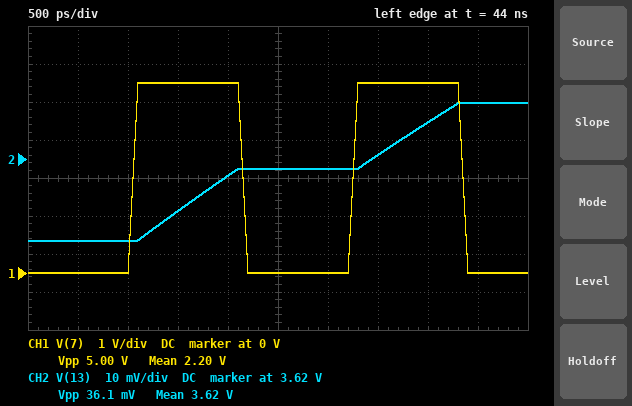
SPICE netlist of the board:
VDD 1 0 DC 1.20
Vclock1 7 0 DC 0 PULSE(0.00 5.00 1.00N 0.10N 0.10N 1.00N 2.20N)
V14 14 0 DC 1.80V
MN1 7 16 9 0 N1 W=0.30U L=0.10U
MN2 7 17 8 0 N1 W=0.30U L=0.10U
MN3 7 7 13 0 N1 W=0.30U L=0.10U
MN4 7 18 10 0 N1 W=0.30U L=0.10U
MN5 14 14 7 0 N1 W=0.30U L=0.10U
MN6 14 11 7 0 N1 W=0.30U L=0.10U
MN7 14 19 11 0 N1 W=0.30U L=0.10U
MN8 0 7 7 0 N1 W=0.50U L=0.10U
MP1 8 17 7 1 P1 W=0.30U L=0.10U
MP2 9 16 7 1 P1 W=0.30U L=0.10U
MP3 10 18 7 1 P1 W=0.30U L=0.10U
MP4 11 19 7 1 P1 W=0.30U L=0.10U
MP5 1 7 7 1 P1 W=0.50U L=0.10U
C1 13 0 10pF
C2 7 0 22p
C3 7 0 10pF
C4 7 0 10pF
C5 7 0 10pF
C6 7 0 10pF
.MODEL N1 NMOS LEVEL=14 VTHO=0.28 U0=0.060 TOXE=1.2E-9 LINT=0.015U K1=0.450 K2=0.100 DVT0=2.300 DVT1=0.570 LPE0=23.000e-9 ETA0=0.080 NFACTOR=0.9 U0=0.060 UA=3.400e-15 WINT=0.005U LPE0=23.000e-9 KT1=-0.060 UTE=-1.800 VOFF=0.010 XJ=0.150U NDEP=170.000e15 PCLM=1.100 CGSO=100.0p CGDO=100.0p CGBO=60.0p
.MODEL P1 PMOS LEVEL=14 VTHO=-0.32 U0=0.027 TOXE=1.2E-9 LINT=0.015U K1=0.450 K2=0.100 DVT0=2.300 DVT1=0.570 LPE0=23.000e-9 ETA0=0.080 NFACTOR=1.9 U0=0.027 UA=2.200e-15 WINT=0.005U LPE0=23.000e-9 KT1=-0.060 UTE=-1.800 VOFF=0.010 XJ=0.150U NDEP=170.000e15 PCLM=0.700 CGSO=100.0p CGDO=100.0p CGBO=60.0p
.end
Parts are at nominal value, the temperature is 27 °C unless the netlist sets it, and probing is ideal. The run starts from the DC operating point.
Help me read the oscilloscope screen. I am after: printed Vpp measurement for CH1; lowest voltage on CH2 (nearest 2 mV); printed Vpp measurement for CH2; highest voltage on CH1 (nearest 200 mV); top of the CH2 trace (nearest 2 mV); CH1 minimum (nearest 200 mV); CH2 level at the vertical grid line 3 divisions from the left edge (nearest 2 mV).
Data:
5.00 V
3.598 V
36.1 mV
5.0 V
3.634 V
0 V
3.606 V
